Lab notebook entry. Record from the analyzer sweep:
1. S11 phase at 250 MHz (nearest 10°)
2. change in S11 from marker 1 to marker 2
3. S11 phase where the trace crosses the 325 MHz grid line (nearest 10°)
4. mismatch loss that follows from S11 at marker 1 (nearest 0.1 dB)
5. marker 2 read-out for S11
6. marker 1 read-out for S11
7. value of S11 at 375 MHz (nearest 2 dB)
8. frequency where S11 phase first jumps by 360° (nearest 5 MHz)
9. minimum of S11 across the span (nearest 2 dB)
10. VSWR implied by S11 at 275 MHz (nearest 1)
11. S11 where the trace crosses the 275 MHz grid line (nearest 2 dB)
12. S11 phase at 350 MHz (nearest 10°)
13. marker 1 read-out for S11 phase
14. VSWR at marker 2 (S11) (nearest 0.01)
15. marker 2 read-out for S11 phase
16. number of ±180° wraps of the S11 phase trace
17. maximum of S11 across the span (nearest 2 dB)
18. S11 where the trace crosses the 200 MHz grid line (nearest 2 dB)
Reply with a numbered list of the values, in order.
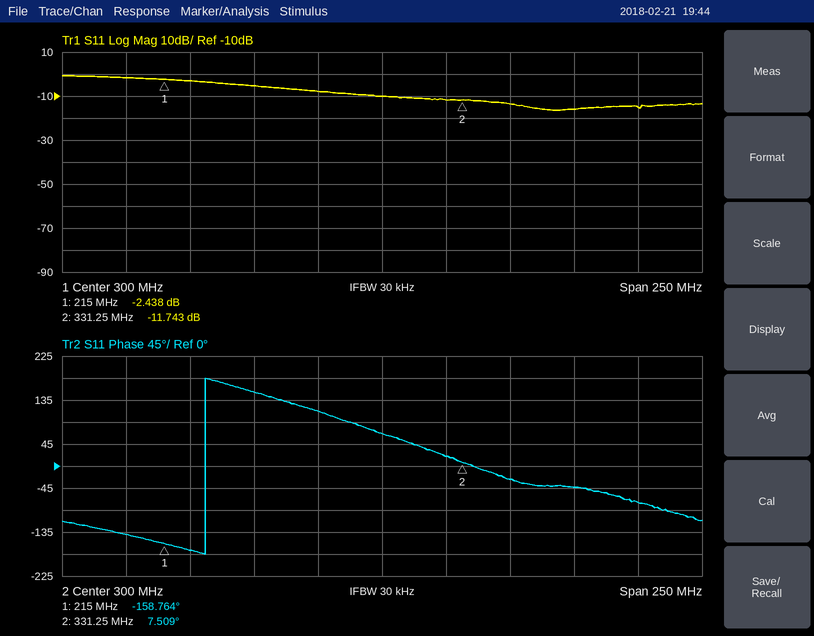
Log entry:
1. 150°
2. -9.305 dB
3. 20°
4. 3.7 dB
5. -11.743 dB
6. -2.438 dB
7. -16 dB
8. 230 MHz
9. -16 dB
10. 2
11. -8 dB
12. -30°
13. -158.764°
14. 1.70
15. 7.509°
16. 1
17. 0 dB
18. -2 dB
